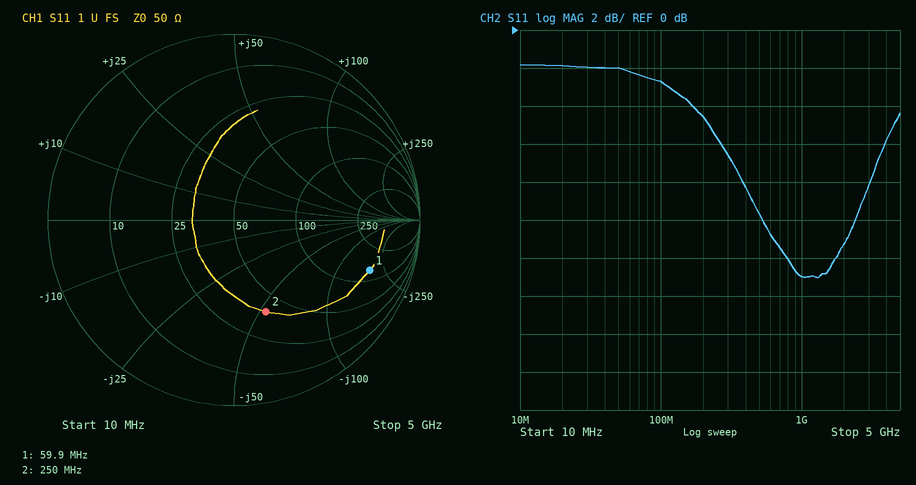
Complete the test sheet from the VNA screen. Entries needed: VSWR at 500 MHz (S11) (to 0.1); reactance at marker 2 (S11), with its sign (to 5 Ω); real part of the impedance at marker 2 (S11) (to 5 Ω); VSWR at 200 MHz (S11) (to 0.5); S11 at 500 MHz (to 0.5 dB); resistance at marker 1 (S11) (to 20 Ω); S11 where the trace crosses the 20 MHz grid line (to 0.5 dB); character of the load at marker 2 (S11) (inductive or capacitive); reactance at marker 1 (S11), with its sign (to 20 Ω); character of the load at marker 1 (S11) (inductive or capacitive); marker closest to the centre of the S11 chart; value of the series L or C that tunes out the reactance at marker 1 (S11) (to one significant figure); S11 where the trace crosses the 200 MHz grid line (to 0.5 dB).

2.0
-55 Ω
40 Ω
4.0
-9.5 dB
140 Ω
-2.0 dB
capacitive
-180 Ω
capacitive
marker 2
500 nH
-4.5 dB
